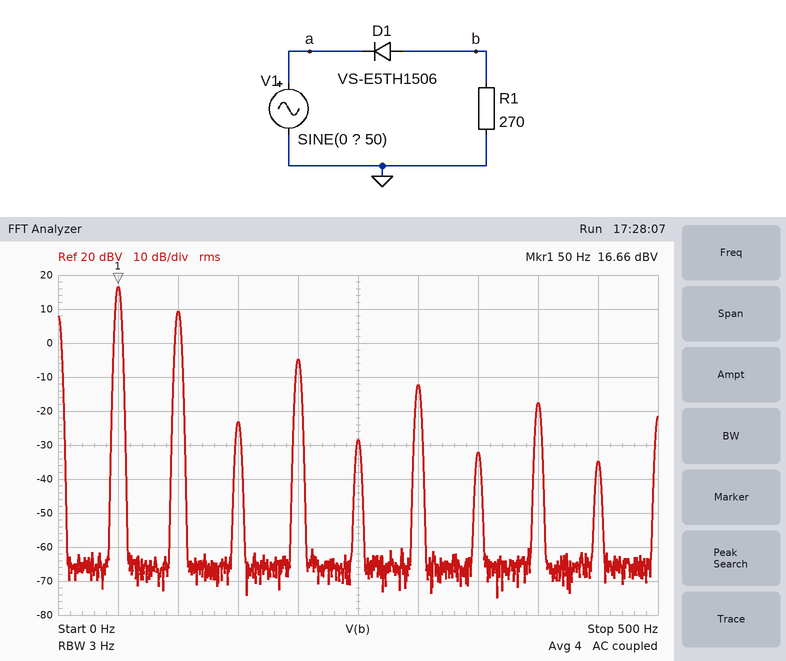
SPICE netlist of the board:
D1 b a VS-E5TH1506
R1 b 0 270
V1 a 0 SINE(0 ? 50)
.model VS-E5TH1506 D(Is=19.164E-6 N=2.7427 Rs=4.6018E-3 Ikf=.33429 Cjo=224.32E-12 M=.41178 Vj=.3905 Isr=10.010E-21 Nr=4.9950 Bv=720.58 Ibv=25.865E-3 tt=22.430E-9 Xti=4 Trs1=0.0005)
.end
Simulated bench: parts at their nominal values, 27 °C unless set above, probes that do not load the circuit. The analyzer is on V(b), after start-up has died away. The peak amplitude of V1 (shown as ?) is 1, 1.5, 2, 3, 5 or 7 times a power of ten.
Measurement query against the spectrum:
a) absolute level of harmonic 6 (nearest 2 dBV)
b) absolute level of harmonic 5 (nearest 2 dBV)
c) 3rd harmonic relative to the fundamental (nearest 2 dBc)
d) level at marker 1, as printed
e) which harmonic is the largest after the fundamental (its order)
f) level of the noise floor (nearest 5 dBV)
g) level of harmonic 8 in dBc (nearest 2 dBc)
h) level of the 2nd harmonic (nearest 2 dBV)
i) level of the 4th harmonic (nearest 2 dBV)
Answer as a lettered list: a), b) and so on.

a) -12 dBV
b) -28 dBV
c) -40 dBc
d) 16.66 dBV
e) 2
f) -65 dBV
g) -34 dBc
h) 10 dBV
i) -4 dBV
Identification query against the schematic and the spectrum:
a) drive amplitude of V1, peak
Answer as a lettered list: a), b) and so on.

a) 20 V
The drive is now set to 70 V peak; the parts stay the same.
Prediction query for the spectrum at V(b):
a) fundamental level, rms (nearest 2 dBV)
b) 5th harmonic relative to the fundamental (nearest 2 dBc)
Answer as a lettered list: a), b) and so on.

a) 28 dBV
b) -54 dBc
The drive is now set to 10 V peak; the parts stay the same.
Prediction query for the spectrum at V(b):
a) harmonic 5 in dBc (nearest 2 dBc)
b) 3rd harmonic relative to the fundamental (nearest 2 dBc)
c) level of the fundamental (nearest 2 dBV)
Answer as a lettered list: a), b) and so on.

a) -40 dBc
b) -34 dBc
c) 10 dBV
